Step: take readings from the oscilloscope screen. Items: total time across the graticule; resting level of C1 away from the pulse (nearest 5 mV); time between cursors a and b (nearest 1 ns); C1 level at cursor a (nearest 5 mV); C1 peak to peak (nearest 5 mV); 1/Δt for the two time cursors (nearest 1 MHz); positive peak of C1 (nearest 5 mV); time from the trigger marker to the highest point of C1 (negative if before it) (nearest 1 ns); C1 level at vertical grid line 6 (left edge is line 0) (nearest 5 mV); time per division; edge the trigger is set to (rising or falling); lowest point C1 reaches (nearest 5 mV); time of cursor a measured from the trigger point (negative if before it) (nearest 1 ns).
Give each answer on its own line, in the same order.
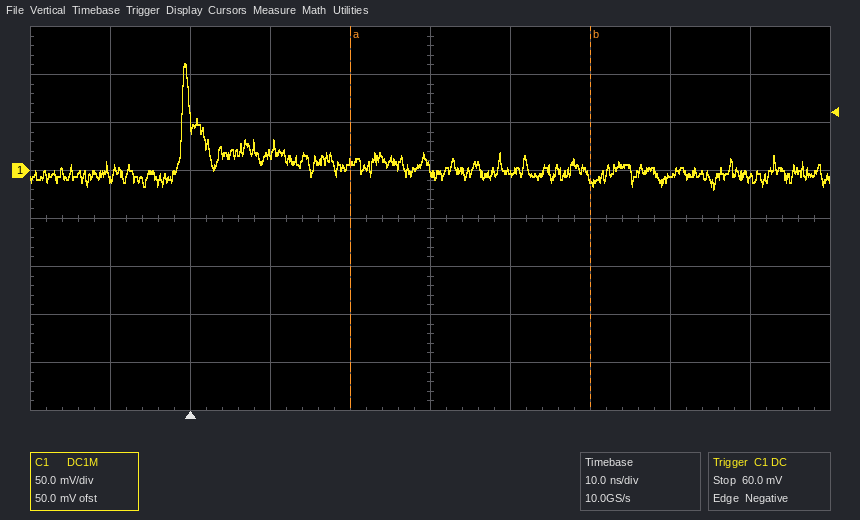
100 ns
0 mV
30 ns
10 mV
130 mV
33 MHz
110 mV
-1 ns
0 mV
10 ns
falling
-20 mV
+20 ns
